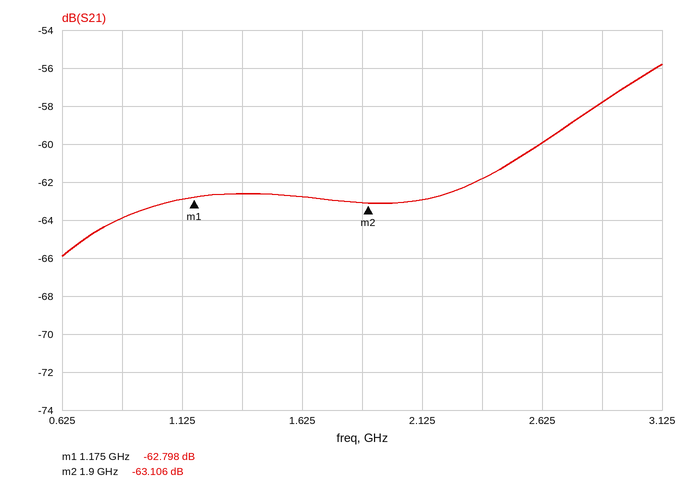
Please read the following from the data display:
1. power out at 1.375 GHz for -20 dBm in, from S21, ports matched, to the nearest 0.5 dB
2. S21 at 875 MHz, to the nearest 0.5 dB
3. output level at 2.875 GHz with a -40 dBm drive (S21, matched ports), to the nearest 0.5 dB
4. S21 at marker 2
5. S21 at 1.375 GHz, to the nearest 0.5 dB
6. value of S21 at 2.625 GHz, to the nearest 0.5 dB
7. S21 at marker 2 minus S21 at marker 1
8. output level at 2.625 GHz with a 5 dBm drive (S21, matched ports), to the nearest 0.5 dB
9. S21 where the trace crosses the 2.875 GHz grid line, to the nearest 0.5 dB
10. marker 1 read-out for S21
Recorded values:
-82.5 dBm
-64.0 dB
-98.0 dBm
-63.106 dB
-62.5 dB
-60.0 dB
-0.308 dB
-55.0 dBm
-58.0 dB
-62.798 dB
